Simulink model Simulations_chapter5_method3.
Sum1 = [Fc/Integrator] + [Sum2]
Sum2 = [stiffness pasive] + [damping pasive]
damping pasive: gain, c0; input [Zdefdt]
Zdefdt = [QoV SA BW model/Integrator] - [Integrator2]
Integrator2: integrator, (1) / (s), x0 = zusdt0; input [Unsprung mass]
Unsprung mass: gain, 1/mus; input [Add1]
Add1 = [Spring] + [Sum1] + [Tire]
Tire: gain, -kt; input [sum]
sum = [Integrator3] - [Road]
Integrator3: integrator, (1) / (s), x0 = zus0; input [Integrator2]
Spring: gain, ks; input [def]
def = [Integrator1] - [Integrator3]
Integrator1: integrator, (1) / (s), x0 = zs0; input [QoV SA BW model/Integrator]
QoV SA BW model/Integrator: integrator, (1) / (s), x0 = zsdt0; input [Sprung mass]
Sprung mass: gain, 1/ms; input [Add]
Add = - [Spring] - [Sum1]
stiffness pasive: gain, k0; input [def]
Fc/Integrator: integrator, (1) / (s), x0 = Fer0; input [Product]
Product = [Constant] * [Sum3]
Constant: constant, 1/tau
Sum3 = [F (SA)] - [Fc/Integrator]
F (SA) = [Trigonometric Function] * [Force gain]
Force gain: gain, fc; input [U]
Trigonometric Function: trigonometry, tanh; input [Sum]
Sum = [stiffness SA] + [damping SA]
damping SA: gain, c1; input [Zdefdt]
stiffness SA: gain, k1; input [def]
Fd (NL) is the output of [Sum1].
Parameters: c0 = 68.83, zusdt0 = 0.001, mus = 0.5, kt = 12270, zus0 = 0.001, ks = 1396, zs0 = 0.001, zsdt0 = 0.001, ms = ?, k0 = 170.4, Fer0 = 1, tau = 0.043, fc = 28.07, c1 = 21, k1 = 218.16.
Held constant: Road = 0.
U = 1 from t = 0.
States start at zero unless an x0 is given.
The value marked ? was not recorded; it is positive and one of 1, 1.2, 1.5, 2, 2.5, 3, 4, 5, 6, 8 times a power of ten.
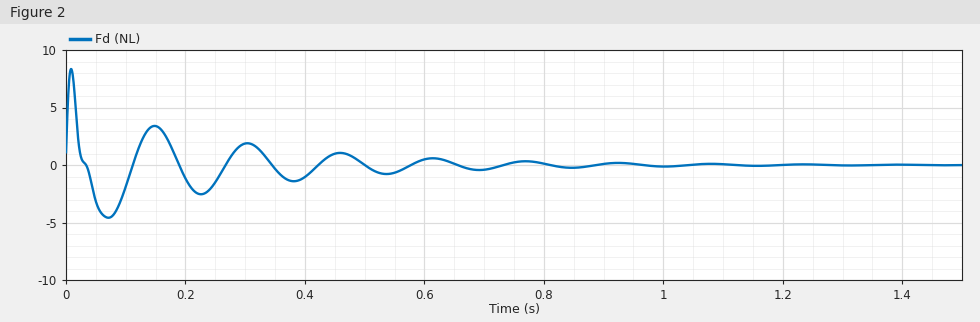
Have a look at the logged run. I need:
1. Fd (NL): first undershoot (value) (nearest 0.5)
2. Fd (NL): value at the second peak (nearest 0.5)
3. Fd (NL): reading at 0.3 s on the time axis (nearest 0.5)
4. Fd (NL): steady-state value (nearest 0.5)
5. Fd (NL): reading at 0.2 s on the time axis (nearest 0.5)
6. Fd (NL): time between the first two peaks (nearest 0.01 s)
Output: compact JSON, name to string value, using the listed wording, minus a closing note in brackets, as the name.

{"Fd (NL): first undershoot (value)": "-4.5", "Fd (NL): value at the second peak": "3.5", "Fd (NL): reading at 0.3 s on the time axis": "2.0", "Fd (NL): steady-state value": "0.0", "Fd (NL): reading at 0.2 s on the time axis": "-1.0", "Fd (NL): time between the first two peaks": "0.14 s"}
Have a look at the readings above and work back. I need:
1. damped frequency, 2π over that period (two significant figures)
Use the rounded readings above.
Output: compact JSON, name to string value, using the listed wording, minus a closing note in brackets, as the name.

{"damped frequency, 2π over that period": "45 rad/s"}
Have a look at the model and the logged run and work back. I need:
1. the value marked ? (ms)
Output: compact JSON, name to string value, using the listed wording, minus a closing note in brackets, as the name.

{"the value marked ?": "4"}
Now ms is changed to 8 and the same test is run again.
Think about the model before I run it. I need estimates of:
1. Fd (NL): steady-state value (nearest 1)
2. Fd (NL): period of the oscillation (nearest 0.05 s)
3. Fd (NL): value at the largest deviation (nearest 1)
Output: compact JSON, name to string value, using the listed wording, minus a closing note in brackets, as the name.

{"Fd (NL): steady-state value": "0", "Fd (NL): period of the oscillation": "0.20 s", "Fd (NL): value at the largest deviation": "9"}
